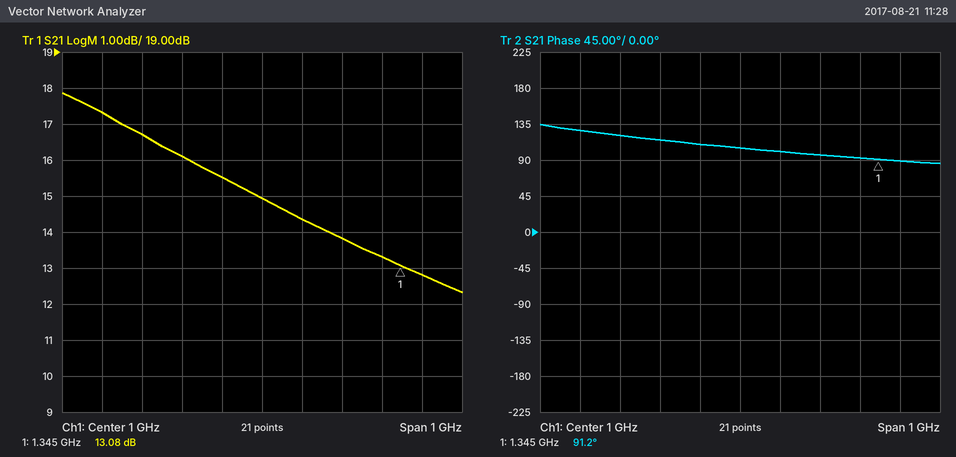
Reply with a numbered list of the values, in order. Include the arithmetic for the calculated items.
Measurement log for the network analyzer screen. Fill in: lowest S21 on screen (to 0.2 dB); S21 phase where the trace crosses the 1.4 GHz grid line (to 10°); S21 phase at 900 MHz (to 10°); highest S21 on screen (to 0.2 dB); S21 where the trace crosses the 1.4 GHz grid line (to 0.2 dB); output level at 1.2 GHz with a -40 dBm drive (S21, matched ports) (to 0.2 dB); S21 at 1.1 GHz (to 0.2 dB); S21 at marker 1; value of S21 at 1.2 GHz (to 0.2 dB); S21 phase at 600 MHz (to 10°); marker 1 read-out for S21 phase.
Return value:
1. 12.4 dB
2. 90°
3. 110°
4. 17.8 dB
5. 12.8 dB
6. -40 dBm + (13.8 dB) = -26.2 dBm
7. 14.4 dB
8. 13.08 dB
9. 13.8 dB
10. 130°
11. 91.2°
